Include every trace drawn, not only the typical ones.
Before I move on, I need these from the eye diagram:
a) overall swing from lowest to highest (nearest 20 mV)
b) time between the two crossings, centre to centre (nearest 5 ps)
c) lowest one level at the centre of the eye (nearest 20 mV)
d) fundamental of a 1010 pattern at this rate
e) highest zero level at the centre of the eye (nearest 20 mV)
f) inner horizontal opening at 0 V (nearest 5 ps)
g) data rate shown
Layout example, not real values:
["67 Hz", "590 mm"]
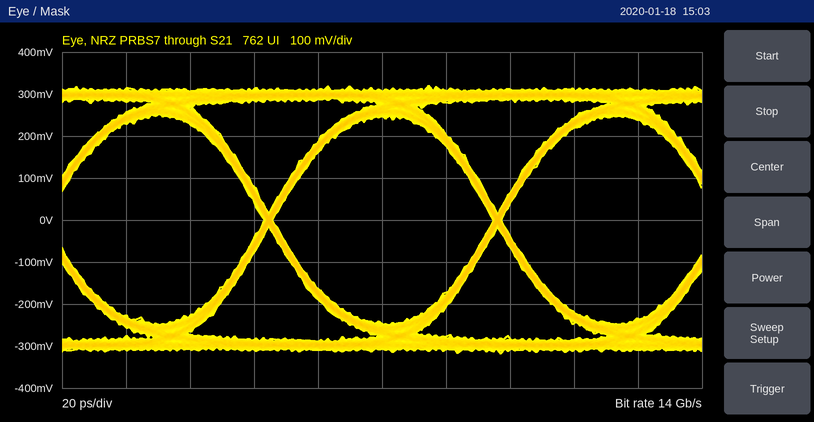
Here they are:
["640 mV", "70 ps", "240 mV", "7 GHz", "-240 mV", "70 ps", "14 Gb/s"]
